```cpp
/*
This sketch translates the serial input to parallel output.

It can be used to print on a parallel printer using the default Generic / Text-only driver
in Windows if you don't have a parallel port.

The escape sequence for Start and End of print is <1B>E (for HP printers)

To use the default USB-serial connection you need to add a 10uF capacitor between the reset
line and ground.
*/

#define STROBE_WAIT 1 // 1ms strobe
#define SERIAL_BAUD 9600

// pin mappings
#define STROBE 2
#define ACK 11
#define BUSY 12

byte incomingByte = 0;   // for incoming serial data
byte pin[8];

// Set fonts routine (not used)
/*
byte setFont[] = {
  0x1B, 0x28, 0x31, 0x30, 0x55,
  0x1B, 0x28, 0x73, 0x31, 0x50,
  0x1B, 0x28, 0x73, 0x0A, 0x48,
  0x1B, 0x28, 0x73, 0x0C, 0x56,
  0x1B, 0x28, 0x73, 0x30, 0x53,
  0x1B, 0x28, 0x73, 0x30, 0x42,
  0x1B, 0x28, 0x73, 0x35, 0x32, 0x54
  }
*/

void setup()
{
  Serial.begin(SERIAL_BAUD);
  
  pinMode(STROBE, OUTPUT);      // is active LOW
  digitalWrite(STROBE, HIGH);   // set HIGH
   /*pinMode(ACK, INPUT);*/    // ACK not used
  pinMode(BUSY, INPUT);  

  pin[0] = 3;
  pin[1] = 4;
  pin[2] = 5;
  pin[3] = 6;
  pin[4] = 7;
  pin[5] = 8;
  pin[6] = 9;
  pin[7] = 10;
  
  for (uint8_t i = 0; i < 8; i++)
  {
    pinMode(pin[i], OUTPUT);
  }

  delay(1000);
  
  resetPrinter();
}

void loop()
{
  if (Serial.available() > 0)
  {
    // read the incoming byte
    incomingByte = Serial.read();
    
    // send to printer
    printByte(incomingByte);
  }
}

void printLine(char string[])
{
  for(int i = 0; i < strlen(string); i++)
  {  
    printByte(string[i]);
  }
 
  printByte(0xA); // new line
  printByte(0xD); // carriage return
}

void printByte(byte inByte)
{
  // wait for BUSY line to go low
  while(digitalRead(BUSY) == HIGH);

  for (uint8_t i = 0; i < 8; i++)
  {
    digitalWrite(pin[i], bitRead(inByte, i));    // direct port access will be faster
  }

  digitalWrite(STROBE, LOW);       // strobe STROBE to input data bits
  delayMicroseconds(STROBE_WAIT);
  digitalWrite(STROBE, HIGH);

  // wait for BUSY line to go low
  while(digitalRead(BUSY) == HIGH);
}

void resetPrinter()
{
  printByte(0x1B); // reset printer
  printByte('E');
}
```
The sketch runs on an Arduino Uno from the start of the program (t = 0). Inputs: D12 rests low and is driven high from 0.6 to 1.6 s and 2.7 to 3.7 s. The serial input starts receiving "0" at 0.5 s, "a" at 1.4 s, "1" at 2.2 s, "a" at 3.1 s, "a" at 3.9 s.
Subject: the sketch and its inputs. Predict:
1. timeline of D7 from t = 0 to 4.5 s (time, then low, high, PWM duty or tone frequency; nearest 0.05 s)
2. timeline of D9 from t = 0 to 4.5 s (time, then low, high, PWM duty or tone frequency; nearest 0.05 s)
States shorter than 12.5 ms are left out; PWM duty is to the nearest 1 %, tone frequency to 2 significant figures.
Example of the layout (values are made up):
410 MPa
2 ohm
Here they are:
0 s low; 2.2 s high; 3.7 s low
0 s low; 1.6 s high; 2.2 s low; 3.7 s high
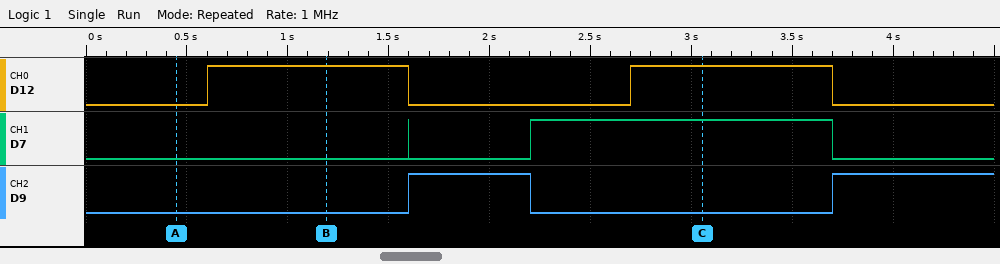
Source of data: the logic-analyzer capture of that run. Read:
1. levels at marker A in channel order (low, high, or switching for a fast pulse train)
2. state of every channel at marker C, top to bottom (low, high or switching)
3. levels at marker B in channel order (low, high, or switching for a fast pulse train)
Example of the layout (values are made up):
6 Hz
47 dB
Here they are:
D12 low, D7 low, D9 low
D12 high, D7 high, D9 low
D12 high, D7 low, D9 low
